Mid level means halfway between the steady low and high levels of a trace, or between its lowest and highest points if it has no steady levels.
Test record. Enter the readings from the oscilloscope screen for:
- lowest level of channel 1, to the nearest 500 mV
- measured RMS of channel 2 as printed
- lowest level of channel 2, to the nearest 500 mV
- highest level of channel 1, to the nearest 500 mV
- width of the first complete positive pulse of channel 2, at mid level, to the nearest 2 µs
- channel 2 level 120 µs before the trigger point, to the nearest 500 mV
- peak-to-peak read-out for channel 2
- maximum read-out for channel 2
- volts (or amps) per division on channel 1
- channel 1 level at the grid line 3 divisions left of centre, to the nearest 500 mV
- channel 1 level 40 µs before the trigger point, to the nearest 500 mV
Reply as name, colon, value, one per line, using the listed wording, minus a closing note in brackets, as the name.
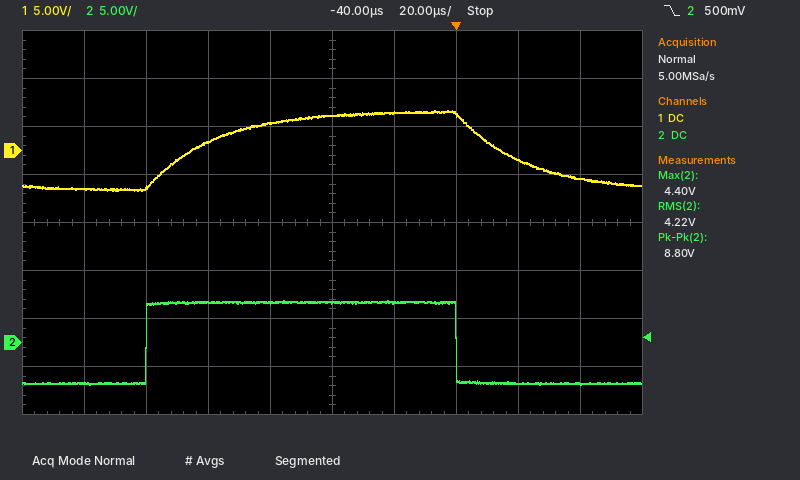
lowest level of channel 1, to the nearest 500 mV: -4.0 V
measured RMS of channel 2 as printed: 4.22 V
lowest level of channel 2, to the nearest 500 mV: -4.5 V
highest level of channel 1, to the nearest 500 mV: 4.0 V
width of the first complete positive pulse of channel 2, at mid level, to the nearest 2 µs: 100 µs
channel 2 level 120 µs before the trigger point, to the nearest 500 mV: -4.0 V
peak-to-peak read-out for channel 2: 8.80 V
maximum read-out for channel 2: 4.40 V
volts (or amps) per division on channel 1: 5 V
channel 1 level at the grid line 3 divisions left of centre, to the nearest 500 mV: -4.0 V
channel 1 level 40 µs before the trigger point, to the nearest 500 mV: 3.5 V
